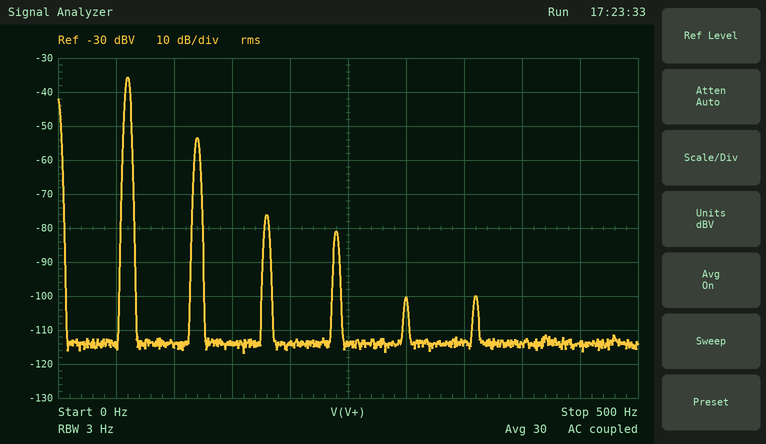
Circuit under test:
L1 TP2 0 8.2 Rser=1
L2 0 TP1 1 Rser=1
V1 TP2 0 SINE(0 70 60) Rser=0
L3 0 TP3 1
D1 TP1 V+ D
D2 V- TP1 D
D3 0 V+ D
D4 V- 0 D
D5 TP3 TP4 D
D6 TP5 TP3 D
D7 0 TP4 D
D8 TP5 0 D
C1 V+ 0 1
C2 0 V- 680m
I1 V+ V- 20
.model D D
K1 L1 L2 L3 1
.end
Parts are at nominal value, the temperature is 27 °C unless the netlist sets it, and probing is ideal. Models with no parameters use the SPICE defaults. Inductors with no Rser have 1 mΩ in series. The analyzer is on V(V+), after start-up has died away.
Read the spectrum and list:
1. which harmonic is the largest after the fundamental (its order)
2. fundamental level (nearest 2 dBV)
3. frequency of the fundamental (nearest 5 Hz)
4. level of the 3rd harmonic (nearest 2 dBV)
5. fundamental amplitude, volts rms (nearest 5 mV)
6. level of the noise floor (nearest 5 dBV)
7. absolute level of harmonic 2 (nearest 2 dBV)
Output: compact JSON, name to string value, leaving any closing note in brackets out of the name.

{"which harmonic is the largest after the fundamental": "2", "fundamental level": "-36 dBV", "frequency of the fundamental": "60 Hz", "level of the 3rd harmonic": "-76 dBV", "fundamental amplitude, volts rms": "15 mV", "level of the noise floor": "-115 dBV", "absolute level of harmonic 2": "-54 dBV"}
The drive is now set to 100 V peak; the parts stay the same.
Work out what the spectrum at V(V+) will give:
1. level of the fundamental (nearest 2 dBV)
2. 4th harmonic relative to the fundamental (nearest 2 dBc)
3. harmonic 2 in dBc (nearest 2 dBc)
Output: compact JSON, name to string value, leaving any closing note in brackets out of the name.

{"level of the fundamental": "-32 dBV", "4th harmonic relative to the fundamental": "-38 dBc", "harmonic 2 in dBc": "-16 dBc"}
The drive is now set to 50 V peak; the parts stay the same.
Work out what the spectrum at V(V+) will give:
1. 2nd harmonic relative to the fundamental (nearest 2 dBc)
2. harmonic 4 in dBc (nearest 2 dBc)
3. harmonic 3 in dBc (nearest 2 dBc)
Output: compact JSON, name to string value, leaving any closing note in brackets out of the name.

{"2nd harmonic relative to the fundamental": "-20 dBc", "harmonic 4 in dBc": "-54 dBc", "harmonic 3 in dBc": "-44 dBc"}
